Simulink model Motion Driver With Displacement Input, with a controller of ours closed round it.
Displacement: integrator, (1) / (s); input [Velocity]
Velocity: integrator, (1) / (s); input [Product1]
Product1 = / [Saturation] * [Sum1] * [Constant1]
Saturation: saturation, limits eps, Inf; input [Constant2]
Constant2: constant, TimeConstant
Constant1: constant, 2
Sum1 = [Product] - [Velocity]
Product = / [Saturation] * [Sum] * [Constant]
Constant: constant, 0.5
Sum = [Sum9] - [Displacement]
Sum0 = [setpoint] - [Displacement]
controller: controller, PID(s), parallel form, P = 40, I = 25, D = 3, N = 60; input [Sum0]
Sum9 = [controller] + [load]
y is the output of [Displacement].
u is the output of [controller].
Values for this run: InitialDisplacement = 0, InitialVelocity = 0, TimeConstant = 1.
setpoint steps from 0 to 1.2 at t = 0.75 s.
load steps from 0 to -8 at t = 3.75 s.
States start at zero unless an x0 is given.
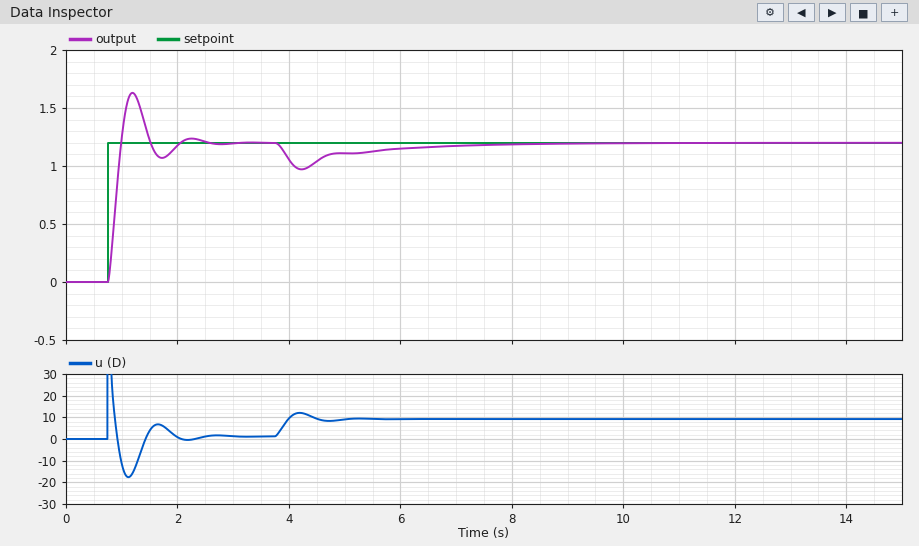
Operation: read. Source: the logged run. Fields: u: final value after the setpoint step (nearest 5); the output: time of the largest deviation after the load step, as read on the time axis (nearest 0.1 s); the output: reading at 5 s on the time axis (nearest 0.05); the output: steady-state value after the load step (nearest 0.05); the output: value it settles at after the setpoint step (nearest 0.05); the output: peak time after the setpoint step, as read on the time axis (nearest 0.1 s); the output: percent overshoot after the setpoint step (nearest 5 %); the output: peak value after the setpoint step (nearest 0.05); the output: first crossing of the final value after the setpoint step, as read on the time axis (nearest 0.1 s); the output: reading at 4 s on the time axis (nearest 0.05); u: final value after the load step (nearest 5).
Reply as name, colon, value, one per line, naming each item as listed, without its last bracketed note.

u: final value after the setpoint step: 0
the output: time of the largest deviation after the load step, as read on the time axis: 4.2 s
the output: reading at 5 s on the time axis: 1.10
the output: steady-state value after the load step: 1.20
the output: value it settles at after the setpoint step: 1.20
the output: peak time after the setpoint step, as read on the time axis: 1.2 s
the output: percent overshoot after the setpoint step: 35 %
the output: peak value after the setpoint step: 1.65
the output: first crossing of the final value after the setpoint step, as read on the time axis: 1.0 s
the output: reading at 4 s on the time axis: 1.05
u: final value after the load step: 10
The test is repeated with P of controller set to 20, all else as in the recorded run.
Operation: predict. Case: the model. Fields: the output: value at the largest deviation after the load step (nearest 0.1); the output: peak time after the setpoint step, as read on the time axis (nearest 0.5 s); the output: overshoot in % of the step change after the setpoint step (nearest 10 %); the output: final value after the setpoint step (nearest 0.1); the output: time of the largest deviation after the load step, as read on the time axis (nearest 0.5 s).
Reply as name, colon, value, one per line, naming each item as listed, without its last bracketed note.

the output: value at the largest deviation after the load step: 0.8
the output: peak time after the setpoint step, as read on the time axis: 1.5 s
the output: overshoot in % of the step change after the setpoint step: 30 %
the output: final value after the setpoint step: 1.2
the output: time of the largest deviation after the load step, as read on the time axis: 4.5 s
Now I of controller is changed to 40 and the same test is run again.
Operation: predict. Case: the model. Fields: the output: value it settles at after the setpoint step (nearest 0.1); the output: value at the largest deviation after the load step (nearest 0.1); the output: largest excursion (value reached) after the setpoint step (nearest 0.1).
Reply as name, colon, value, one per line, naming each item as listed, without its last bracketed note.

the output: value it settles at after the setpoint step: 1.2
the output: value at the largest deviation after the load step: 1.0
the output: largest excursion (value reached) after the setpoint step: 1.7
